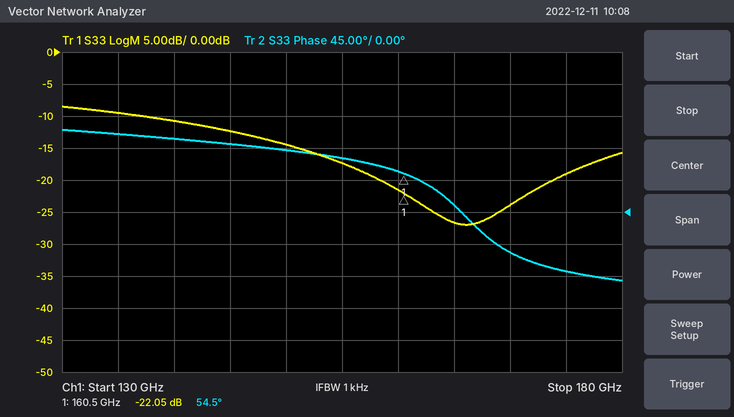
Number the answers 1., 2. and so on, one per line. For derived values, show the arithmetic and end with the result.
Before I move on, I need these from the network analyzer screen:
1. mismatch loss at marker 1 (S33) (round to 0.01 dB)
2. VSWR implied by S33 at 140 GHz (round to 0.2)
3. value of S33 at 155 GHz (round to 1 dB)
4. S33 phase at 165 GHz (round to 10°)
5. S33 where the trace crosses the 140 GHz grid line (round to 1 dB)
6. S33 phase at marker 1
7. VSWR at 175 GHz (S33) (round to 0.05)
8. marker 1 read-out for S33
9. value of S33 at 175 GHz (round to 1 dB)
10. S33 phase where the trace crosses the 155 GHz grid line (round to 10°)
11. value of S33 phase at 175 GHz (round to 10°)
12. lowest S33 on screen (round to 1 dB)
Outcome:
1. −10 log10(1 − 10^(-22.05/10)) ≈ 0.03 dB
2. |Γ| = 10^(-11/20) = 0.2818; VSWR = (1 + 0.2818)/(1 − 0.2818) ≈ 1.8
3. -17 dB
4. 10°
5. -11 dB
6. 54.5°
7. |Γ| = 10^(-19/20) = 0.1122; VSWR = (1 + 0.1122)/(1 − 0.1122) ≈ 1.25
8. -22.05 dB
9. -19 dB
10. 80°
11. -80°
12. -27 dB
